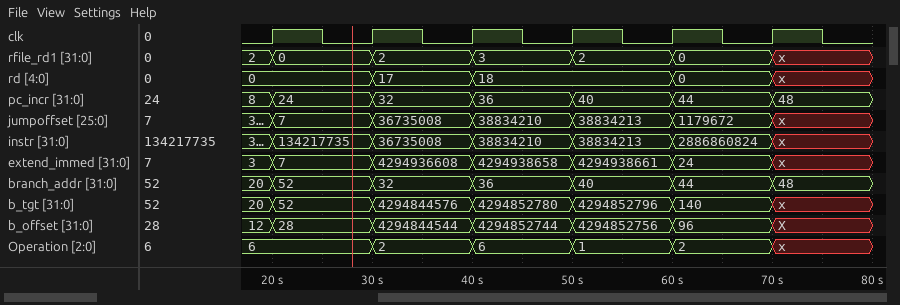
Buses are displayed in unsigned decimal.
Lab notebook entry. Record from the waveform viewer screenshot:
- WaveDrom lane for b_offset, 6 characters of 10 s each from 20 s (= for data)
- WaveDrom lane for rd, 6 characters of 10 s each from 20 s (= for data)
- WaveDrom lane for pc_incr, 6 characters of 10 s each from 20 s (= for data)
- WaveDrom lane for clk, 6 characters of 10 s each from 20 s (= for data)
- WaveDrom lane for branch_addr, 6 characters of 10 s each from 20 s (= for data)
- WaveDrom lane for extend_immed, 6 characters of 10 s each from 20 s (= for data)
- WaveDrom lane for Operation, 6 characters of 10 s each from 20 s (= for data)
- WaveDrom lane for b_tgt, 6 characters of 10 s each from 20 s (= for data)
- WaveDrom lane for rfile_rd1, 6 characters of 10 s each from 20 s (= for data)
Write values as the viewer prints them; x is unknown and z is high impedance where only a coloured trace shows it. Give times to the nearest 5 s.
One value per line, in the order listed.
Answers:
{name: 'b_offset', wave: '======', data: '28 4294844544 4294852744 4294852756 96 X'}
{name: 'rd', wave: '===.=x', data: '0 17 18 0'}
{name: 'pc_incr', wave: '======', data: '24 32 36 40 44 48'}
{name: 'clk', wave: 'p.....'}
{name: 'branch_addr', wave: '======', data: '52 32 36 40 44 48'}
{name: 'extend_immed', wave: '=====x', data: '7 4294936608 4294938658 4294938661 24'}
{name: 'Operation', wave: '=====x', data: '6 2 6 1 2'}
{name: 'b_tgt', wave: '=====x', data: '52 4294844576 4294852780 4294852796 140'}
{name: 'rfile_rd1', wave: '=====x', data: '0 2 3 2 0'}
